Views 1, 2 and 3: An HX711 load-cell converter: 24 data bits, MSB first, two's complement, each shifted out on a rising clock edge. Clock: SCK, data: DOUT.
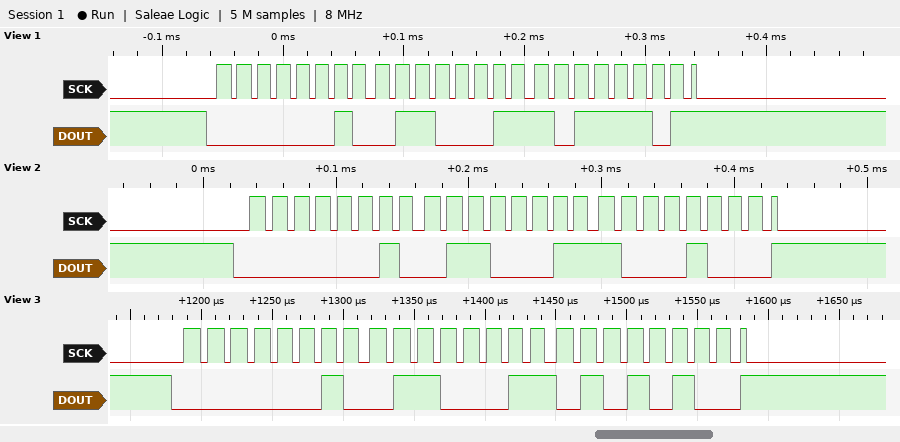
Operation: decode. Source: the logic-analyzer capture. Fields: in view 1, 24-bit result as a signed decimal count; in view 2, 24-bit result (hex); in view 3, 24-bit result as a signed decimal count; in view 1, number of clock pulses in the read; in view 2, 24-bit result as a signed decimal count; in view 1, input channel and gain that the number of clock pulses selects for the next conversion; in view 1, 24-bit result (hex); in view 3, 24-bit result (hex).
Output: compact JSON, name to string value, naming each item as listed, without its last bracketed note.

{"in view 1, 24-bit result as a signed decimal count": "156605", "in view 2, 24-bit result": "0x026388", "in view 3, 24-bit result as a signed decimal count": "156500", "in view 1, number of clock pulses in the read": "25", "in view 2, 24-bit result as a signed decimal count": "156552", "in view 1, input channel and gain that the number of clock pulses selects for the next conversion": "channel A, gain 128", "in view 1, 24-bit result": "0x0263BD", "in view 3, 24-bit result": "0x026354"}
